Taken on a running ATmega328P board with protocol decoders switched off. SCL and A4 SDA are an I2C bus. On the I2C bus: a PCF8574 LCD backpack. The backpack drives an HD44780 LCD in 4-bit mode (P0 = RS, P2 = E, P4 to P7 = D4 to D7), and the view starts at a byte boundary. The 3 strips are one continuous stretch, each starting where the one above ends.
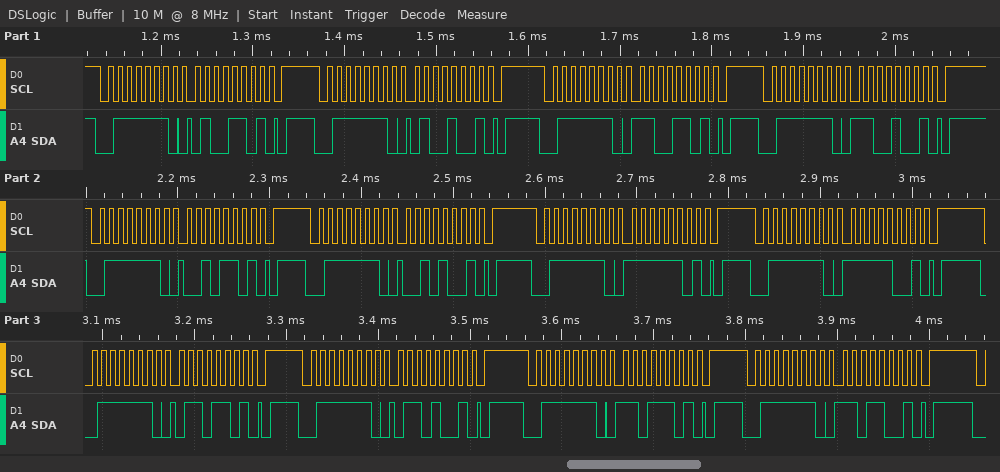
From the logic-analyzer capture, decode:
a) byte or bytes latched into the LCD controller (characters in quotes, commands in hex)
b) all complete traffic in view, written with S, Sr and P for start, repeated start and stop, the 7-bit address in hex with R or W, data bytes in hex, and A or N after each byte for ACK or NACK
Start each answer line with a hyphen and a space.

- 'L' '/' 'm'
- S 3FW A 4D A P S 3FW A 49 A P S 3FW A CD A P S 3FW A C9 A P S 3FW A 2D A P S 3FW A 29 A P S 3FW A FD A P S 3FW A F9 A P S 3FW A 6D A P S 3FW A 69 A P S 3FW A DD A P S 3FW A D9 A P
